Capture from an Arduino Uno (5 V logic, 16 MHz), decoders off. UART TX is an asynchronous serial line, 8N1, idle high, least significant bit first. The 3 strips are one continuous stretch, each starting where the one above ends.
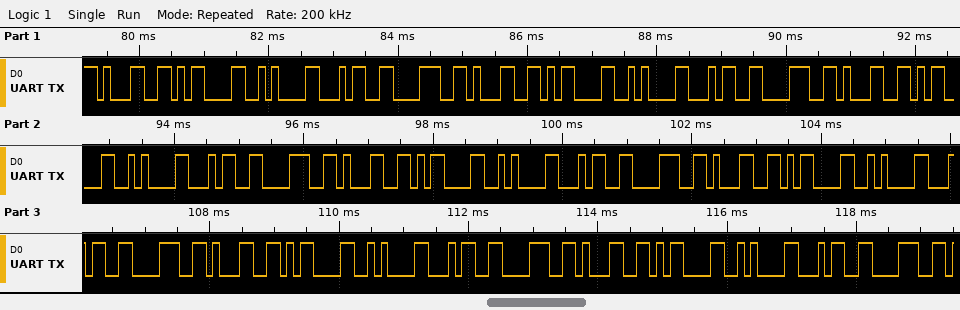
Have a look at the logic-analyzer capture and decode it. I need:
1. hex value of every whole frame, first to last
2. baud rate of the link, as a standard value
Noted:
31 0D 0A 34 38 31 0D 0A 34 38 31 0D 0A 34 38 31 0D 0A 34 38 31 0D 0A 34 38 31 0D 0A 34 38 31 0D 0A 34 38
9600 baud
